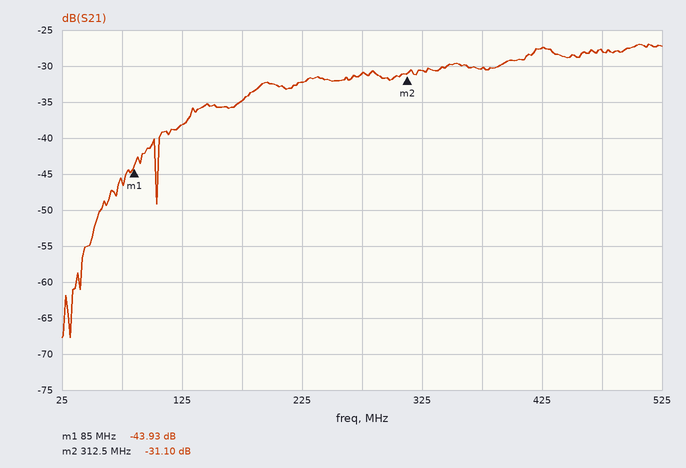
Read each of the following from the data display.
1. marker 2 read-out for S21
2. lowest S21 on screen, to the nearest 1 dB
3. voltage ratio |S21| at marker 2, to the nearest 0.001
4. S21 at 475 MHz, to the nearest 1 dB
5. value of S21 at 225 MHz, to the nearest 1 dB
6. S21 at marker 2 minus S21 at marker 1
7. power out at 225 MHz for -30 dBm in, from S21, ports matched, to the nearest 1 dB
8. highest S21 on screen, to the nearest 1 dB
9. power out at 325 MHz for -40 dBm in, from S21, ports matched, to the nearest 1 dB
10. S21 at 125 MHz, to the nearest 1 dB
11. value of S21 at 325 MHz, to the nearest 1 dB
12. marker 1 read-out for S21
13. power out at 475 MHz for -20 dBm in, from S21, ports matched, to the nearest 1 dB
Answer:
-31.10 dB
-68 dB
0.028
-28 dB
-32 dB
12.83 dB
-62 dBm
-27 dB
-71 dBm
-38 dB
-31 dB
-43.93 dB
-48 dBm
